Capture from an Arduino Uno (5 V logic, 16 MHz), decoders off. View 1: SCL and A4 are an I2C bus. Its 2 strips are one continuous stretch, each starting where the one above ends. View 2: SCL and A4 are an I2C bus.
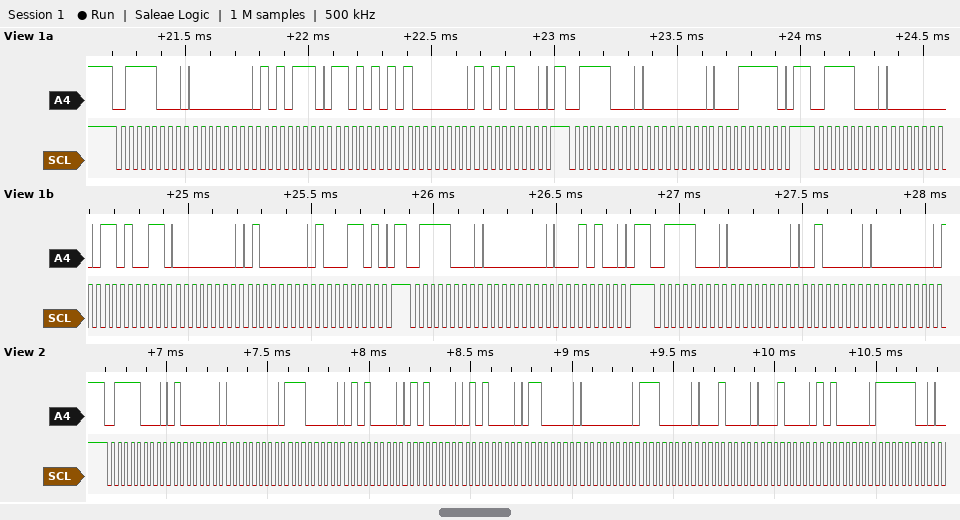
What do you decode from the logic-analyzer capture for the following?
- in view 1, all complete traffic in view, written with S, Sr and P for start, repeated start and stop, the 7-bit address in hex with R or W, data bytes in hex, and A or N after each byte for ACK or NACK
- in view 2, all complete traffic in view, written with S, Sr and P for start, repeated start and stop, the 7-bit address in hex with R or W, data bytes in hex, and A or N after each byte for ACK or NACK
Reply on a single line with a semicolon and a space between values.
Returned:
S 3CW A 00 A AE A D5 A 80 A A8 A P S 3CW A 00 A 1F A P S 3CW A 00 A D3 A 00 A 40 A 8D A P S 3CW A 00 A 14 A P S 3CW A 00 A 20 A 00 A; S 3CW A 40 A 00 A E0 A 50 A 50 A 50 A 60 A 00 A E0 A 10 A 10 A A0 A FC A
